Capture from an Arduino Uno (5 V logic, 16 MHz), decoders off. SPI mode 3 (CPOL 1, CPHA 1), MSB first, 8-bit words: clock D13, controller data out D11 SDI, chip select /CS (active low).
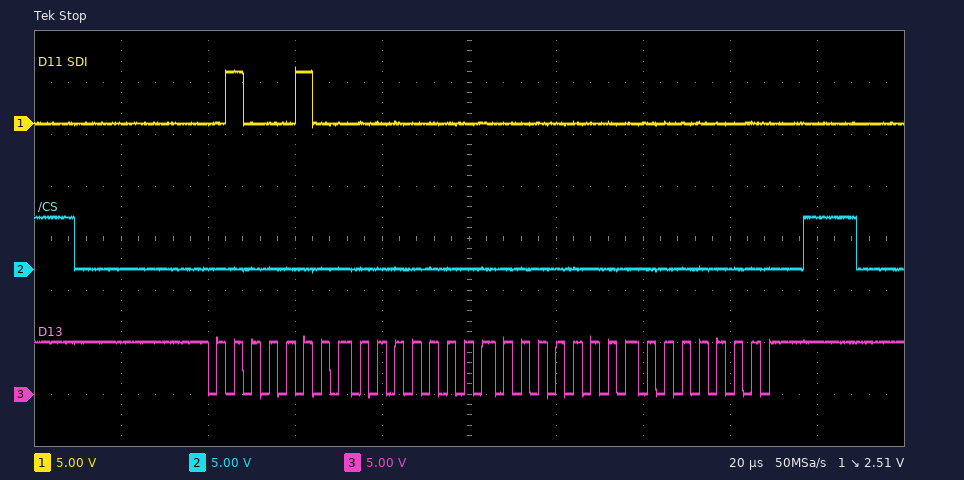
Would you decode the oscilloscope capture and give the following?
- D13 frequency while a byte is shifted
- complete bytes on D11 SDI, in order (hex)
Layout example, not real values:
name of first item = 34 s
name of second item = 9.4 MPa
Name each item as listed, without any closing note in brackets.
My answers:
D13 frequency while a byte is shifted = 250 kHz
complete bytes on D11 SDI, in order = 44 00 00 00
